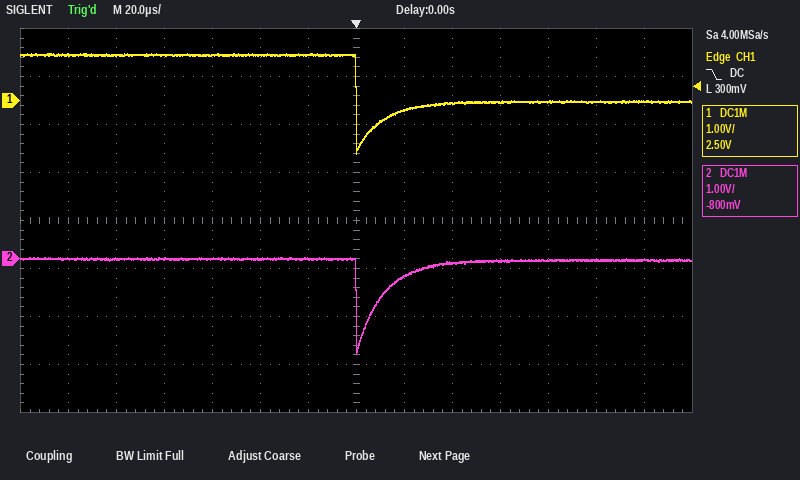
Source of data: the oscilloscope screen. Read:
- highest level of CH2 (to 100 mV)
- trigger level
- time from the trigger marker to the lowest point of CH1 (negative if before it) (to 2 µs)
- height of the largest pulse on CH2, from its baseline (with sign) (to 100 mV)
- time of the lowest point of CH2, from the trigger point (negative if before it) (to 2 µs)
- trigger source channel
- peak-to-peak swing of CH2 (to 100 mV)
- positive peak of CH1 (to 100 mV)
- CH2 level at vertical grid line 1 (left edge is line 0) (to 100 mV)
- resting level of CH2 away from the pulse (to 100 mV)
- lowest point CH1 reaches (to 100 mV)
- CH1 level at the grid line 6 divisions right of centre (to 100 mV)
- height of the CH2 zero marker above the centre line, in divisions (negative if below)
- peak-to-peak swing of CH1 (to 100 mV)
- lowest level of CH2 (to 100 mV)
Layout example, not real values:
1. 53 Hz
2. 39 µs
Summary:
1. 0.0 V
2. 300 mV
3. 0 µs
4. -2.0 V
5. 0 µs
6. CH1
7. 2.0 V
8. 1.0 V
9. 0.0 V
10. 0.0 V
11. -1.1 V
12. 0.0 V
13. -0.8 div
14. 2.1 V
15. -2.0 V
